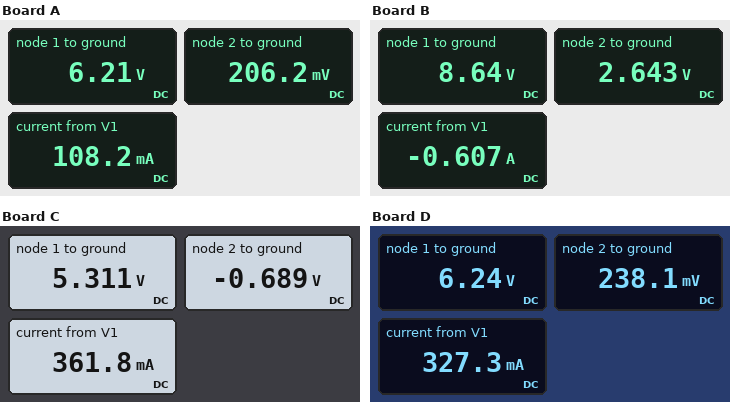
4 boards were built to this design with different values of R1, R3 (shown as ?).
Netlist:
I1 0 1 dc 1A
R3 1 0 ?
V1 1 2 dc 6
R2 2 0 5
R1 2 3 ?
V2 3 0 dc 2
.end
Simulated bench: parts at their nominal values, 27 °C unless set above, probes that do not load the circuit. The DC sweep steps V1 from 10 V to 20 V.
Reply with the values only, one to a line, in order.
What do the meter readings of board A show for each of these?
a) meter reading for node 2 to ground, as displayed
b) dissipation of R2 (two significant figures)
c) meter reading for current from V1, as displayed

206.2 mV
8.5 mW
108.2 mA
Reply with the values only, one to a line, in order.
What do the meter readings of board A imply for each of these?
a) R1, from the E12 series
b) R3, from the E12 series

12 Ω
5.6 Ω
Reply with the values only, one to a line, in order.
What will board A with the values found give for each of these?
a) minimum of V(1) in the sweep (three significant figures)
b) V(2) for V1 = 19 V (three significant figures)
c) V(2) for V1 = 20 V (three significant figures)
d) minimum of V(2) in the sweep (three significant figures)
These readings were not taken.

8.66 V
-4.82 V
-5.21 V
-5.21 V
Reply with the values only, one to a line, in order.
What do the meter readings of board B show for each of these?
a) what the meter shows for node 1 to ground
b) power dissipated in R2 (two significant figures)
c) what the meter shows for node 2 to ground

8.64 V
1.4 W
2.643 V
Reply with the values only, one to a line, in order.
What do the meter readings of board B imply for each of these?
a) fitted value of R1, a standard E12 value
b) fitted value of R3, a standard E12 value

8.2 Ω
22 Ω
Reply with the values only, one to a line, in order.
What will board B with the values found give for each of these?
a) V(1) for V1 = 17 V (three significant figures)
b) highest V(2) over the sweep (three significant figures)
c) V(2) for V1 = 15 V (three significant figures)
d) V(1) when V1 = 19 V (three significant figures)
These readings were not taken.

18.3 V
2.15 V
1.53 V
20.0 V
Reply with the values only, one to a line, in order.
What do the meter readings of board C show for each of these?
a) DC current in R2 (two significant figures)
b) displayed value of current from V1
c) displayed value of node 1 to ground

140 mA
361.8 mA
5.311 V
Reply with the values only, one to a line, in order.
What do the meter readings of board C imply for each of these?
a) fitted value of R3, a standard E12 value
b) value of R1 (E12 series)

3.9 Ω
12 Ω
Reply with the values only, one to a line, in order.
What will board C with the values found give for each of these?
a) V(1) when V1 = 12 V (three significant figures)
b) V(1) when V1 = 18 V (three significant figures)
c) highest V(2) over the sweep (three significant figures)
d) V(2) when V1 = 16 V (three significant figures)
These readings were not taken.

8.46 V
11.6 V
-2.59 V
-5.44 V
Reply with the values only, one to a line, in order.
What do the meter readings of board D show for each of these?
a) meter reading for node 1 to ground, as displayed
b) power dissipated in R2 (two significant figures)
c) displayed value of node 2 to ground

6.24 V
11 mW
238.1 mV
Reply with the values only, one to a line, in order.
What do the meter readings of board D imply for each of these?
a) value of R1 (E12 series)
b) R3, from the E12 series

4.7 Ω
4.7 Ω
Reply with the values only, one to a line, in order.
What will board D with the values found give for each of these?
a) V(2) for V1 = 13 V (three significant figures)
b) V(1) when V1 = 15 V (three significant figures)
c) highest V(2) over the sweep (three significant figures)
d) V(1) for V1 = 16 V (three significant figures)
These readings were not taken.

-2.14 V
12.2 V
-1.12 V
12.8 V
